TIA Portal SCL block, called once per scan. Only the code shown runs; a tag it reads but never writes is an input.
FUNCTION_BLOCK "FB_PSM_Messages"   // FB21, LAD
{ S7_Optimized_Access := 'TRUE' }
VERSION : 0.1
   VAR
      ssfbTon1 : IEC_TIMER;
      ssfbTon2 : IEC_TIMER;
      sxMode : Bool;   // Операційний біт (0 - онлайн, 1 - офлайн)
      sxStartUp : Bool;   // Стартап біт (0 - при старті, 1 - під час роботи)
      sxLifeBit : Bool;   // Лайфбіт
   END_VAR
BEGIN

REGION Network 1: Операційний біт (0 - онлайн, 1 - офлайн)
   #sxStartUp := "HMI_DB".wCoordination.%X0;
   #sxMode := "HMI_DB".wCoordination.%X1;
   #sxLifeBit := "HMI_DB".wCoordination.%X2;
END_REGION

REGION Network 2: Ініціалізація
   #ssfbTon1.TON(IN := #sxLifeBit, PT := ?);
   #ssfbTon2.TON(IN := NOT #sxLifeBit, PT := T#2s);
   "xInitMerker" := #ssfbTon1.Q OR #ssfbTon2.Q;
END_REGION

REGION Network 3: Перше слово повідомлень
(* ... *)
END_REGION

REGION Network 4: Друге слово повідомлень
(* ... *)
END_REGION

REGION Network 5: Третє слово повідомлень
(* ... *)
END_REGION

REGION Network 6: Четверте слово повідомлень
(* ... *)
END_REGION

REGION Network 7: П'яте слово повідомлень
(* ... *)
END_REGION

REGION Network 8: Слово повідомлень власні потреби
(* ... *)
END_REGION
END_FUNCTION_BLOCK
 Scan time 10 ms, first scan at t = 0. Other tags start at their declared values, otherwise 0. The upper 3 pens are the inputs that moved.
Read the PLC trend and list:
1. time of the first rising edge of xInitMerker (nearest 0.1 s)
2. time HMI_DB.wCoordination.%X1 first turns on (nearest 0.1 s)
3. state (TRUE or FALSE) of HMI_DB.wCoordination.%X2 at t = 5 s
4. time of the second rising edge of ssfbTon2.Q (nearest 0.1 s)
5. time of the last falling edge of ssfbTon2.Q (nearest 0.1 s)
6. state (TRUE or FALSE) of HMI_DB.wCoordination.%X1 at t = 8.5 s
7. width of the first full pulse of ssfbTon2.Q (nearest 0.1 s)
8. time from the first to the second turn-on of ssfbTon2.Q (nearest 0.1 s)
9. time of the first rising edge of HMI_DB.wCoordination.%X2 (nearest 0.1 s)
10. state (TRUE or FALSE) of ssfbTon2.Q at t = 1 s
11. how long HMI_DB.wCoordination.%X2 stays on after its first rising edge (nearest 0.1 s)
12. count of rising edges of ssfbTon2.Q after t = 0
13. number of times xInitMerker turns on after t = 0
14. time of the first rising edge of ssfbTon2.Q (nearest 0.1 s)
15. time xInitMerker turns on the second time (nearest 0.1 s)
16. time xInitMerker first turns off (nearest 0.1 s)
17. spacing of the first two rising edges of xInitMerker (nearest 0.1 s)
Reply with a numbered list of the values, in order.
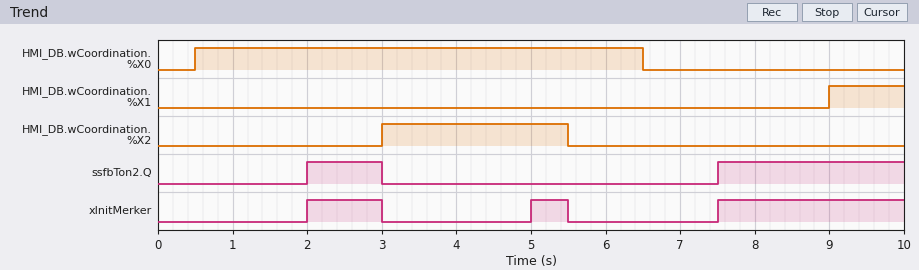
1. 2.0 s
2. 9.0 s
3. TRUE
4. 7.5 s
5. 3.0 s
6. FALSE
7. 1.0 s
8. 5.5 s
9. 3.0 s
10. FALSE
11. 2.5 s
12. 2
13. 3
14. 2.0 s
15. 5.0 s
16. 3.0 s
17. 3.0 s
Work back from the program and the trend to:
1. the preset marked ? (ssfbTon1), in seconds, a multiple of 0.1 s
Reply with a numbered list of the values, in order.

1. 2.0 s
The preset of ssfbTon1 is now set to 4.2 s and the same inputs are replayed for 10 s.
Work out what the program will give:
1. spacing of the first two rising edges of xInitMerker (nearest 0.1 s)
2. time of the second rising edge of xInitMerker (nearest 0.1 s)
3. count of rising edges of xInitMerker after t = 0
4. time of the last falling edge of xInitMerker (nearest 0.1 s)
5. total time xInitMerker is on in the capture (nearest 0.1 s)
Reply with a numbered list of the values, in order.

1. 5.5 s
2. 7.5 s
3. 2
4. 3.0 s
5. 3.5 s
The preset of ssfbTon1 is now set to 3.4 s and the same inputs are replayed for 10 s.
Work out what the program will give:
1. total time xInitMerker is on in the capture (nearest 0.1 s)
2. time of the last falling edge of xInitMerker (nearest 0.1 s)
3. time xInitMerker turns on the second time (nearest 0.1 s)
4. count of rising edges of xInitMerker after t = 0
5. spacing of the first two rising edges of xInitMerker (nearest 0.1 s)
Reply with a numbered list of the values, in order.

1. 3.5 s
2. 3.0 s
3. 7.5 s
4. 2
5. 5.5 s
